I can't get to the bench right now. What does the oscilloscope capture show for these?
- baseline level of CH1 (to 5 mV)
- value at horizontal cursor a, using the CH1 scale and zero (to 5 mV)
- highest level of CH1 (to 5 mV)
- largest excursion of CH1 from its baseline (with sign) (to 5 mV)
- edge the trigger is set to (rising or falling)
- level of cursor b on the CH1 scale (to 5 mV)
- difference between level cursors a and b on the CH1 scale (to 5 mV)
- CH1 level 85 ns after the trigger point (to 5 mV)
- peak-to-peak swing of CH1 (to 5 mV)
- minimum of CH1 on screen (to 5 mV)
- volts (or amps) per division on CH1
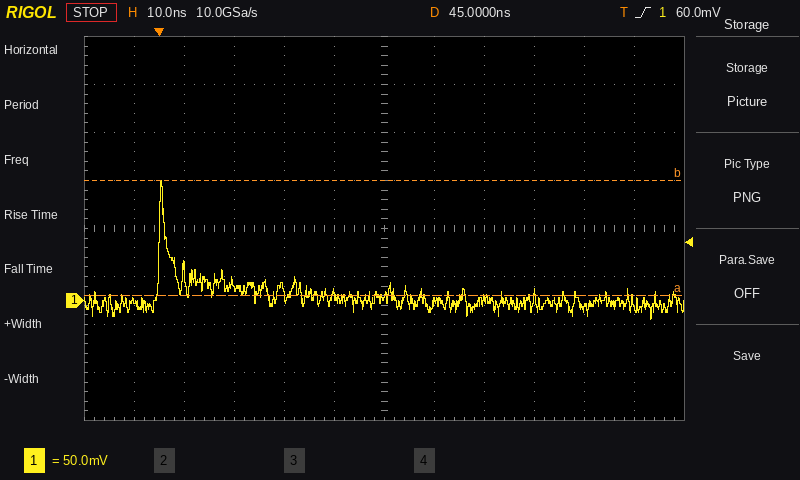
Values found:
0 mV
5 mV
125 mV
+125 mV
rising
125 mV
120 mV
-10 mV
145 mV
-20 mV
50 mV
